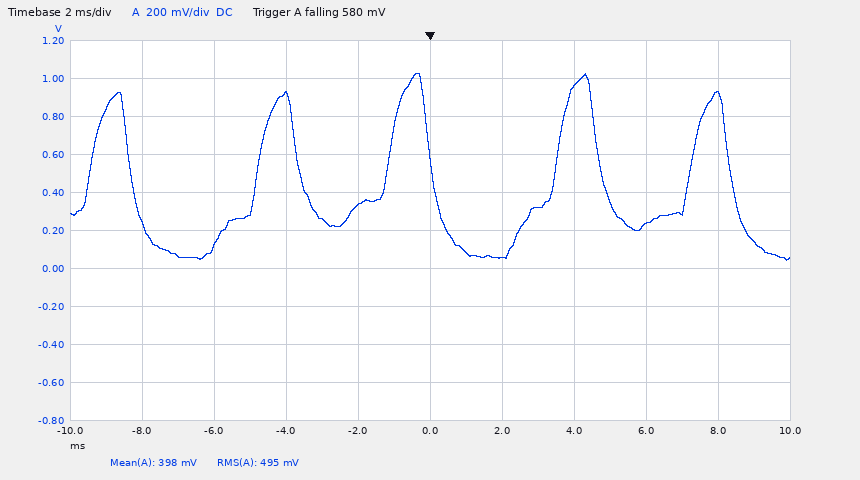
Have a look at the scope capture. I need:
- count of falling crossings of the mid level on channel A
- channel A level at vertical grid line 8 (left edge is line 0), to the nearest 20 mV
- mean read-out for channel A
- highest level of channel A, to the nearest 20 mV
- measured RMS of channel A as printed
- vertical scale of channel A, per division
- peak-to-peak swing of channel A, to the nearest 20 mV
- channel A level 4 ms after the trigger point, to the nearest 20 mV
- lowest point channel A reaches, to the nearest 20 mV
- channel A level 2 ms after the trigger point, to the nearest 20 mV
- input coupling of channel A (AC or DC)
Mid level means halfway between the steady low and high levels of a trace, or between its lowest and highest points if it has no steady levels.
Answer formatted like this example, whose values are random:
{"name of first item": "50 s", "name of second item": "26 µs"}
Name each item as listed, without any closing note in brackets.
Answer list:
{"count of falling crossings of the mid level on channel A": "5", "channel A level at vertical grid line 8 (left edge is line 0), to the nearest 20 mV": "240 mV", "mean read-out for channel A": "398 mV", "highest level of channel A, to the nearest 20 mV": "1.02 V", "measured RMS of channel A as printed": "495 mV", "vertical scale of channel A, per division": "200 mV", "peak-to-peak swing of channel A, to the nearest 20 mV": "980 mV", "channel A level 4 ms after the trigger point, to the nearest 20 mV": "960 mV", "lowest point channel A reaches, to the nearest 20 mV": "40 mV", "channel A level 2 ms after the trigger point, to the nearest 20 mV": "60 mV", "input coupling of channel A": "DC"}
